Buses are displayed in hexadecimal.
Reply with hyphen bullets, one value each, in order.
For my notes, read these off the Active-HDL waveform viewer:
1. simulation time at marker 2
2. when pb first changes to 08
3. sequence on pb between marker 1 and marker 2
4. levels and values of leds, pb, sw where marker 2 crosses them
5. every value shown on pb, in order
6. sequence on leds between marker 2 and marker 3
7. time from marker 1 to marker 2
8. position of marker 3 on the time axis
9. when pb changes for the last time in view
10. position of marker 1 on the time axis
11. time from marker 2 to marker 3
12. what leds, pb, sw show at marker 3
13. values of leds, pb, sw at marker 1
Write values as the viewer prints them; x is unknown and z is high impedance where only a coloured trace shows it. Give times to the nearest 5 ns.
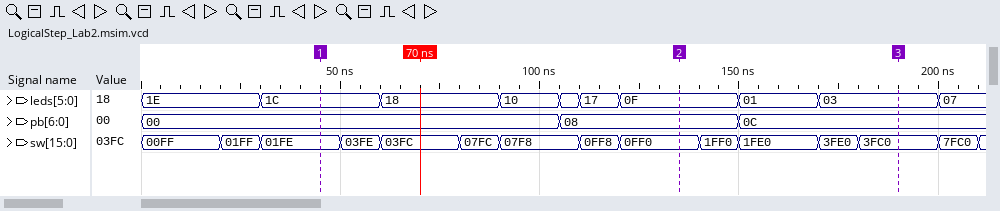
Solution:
- 135 ns
- 105 ns
- 00, 08
- leds=0F, pb=08, sw=0FF0
- 00, 08, 0C
- 0F, 01, 03
- 90 ns
- 190 ns
- 150 ns
- 45 ns
- 55 ns
- leds=03, pb=0C, sw=3FC0
- leds=1C, pb=00, sw=01FE
